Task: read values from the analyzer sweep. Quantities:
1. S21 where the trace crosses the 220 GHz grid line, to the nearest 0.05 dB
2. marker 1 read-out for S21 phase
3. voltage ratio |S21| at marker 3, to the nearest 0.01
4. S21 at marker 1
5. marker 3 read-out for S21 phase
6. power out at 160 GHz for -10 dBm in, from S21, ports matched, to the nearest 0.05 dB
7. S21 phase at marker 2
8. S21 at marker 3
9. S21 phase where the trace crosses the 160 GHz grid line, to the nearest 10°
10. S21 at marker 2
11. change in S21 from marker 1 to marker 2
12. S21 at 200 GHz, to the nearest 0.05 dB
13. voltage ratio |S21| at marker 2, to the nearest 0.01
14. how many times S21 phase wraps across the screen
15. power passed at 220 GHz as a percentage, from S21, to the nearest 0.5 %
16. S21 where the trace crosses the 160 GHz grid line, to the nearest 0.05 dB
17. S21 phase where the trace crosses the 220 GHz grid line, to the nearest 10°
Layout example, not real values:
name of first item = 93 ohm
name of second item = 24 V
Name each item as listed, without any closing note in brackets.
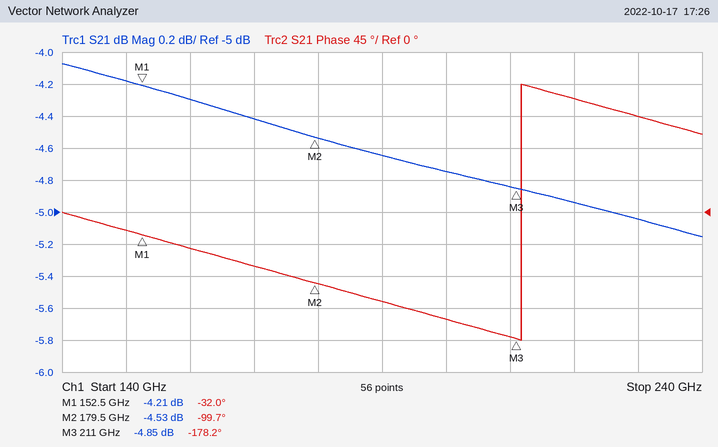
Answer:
S21 where the trace crosses the 220 GHz grid line, to the nearest 0.05 dB = -4.95 dB
marker 1 read-out for S21 phase = -32.0°
voltage ratio |S21| at marker 3, to the nearest 0.01 = 0.57
S21 at marker 1 = -4.21 dB
marker 3 read-out for S21 phase = -178.2°
power out at 160 GHz for -10 dBm in, from S21, ports matched, to the nearest 0.05 dB = -14.30 dBm
S21 phase at marker 2 = -99.7°
S21 at marker 3 = -4.85 dB
S21 phase where the trace crosses the 160 GHz grid line, to the nearest 10° = -50°
S21 at marker 2 = -4.53 dB
change in S21 from marker 1 to marker 2 = -0.32 dB
S21 at 200 GHz, to the nearest 0.05 dB = -4.75 dB
voltage ratio |S21| at marker 2, to the nearest 0.01 = 0.59
how many times S21 phase wraps across the screen = 1
power passed at 220 GHz as a percentage, from S21, to the nearest 0.5 % = 32.0 %
S21 where the trace crosses the 160 GHz grid line, to the nearest 0.05 dB = -4.30 dB
S21 phase where the trace crosses the 220 GHz grid line, to the nearest 10° = 160°
